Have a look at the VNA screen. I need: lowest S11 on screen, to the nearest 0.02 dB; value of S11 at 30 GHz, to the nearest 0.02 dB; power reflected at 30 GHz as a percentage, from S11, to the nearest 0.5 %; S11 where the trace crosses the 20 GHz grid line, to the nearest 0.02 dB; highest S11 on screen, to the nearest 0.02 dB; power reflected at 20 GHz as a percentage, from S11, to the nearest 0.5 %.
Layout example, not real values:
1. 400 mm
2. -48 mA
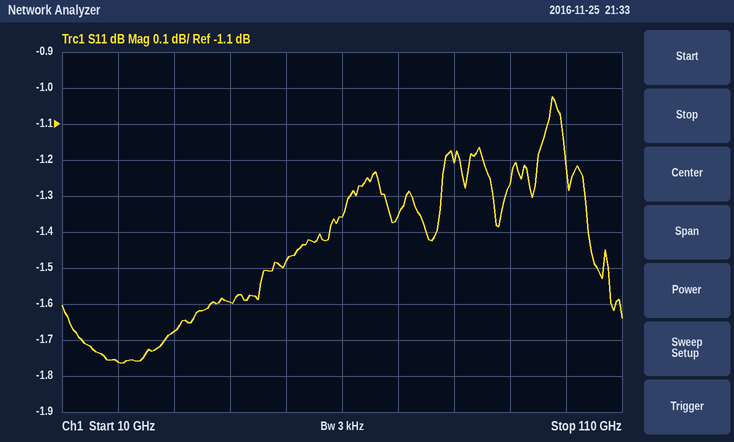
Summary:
1. -1.76 dB
2. -1.68 dB
3. 68.0 %
4. -1.76 dB
5. -1.02 dB
6. 66.5 %
